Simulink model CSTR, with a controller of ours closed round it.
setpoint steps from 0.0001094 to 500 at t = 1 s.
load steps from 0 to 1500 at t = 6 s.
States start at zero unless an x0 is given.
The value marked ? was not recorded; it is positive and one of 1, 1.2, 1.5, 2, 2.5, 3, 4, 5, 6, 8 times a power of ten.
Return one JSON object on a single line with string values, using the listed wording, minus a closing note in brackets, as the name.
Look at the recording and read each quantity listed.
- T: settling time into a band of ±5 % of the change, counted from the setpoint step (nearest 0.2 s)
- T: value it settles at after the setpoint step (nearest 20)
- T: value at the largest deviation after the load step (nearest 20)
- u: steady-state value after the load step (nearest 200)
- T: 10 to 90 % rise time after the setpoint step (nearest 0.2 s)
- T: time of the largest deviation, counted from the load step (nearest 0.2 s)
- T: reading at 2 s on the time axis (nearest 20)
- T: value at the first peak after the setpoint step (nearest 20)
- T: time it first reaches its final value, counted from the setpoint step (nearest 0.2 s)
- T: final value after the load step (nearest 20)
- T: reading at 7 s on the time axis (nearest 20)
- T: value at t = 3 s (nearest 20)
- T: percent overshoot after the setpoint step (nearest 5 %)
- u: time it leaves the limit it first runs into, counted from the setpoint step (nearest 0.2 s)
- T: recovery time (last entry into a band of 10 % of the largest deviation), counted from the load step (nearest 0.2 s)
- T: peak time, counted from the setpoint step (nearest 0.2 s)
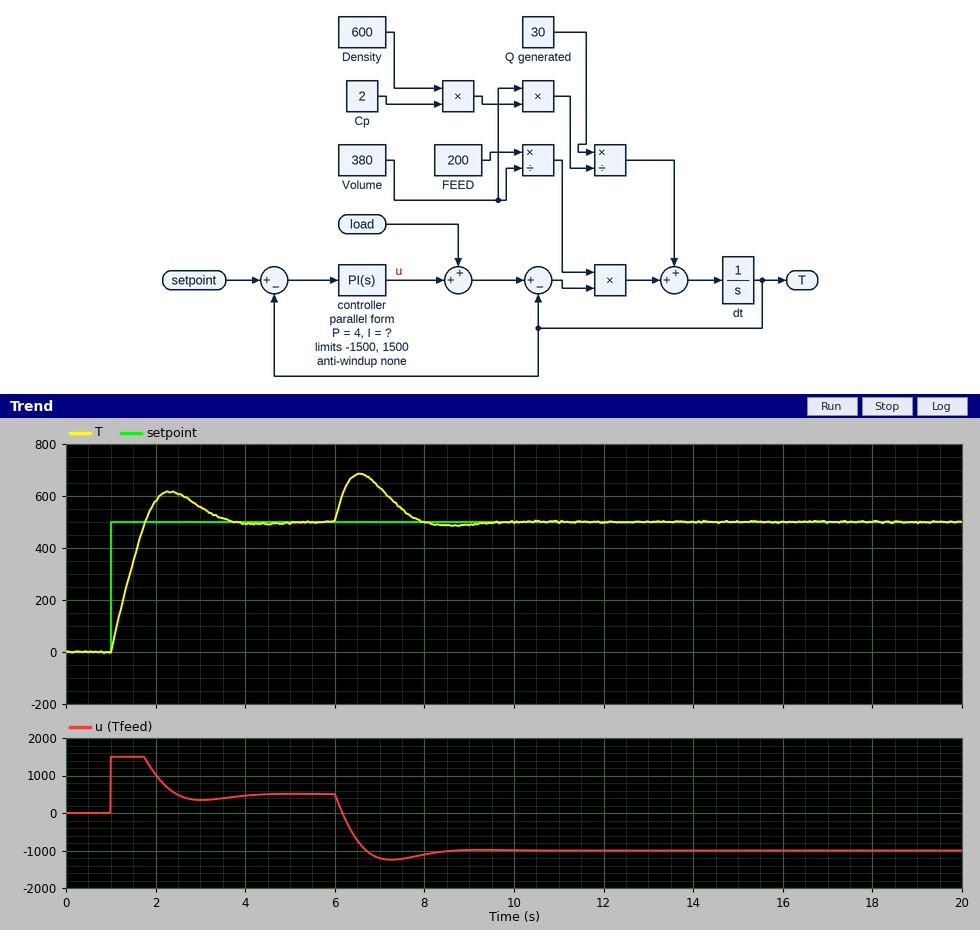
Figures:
{"T: settling time into a band of ±5 % of the change, counted from the setpoint step": "2.4 s", "T: value it settles at after the setpoint step": "500", "T: value at the largest deviation after the load step": "680", "u: steady-state value after the load step": "-1000", "T: 10 to 90 % rise time after the setpoint step": "0.6 s", "T: time of the largest deviation, counted from the load step": "0.6 s", "T: reading at 2 s on the time axis": "580", "T: value at the first peak after the setpoint step": "620", "T: time it first reaches its final value, counted from the setpoint step": "0.8 s", "T: final value after the load step": "500", "T: reading at 7 s on the time axis": "640", "T: value at t = 3 s": "560", "T: percent overshoot after the setpoint step": "25 %", "u: time it leaves the limit it first runs into, counted from the setpoint step": "0.8 s", "T: recovery time (last entry into a band of 10 % of the largest deviation), counted from the load step": "1.8 s", "T: peak time, counted from the setpoint step": "1.4 s"}
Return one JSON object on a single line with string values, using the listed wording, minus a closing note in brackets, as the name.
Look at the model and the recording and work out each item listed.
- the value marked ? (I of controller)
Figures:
{"the value marked ?": "8"}
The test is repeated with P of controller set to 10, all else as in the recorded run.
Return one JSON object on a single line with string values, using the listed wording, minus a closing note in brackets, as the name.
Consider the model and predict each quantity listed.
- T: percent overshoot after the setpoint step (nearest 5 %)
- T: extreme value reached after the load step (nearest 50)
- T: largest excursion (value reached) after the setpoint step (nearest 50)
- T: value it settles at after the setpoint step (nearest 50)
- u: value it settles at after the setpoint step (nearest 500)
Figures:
{"T: percent overshoot after the setpoint step": "15 %", "T: extreme value reached after the load step": "600", "T: largest excursion (value reached) after the setpoint step": "550", "T: value it settles at after the setpoint step": "500", "u: value it settles at after the setpoint step": "500"}
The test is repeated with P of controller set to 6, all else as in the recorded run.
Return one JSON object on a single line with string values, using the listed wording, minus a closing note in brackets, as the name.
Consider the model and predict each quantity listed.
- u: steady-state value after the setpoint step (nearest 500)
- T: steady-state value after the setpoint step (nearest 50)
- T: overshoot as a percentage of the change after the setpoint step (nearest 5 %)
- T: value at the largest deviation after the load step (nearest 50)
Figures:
{"u: steady-state value after the setpoint step": "500", "T: steady-state value after the setpoint step": "500", "T: overshoot as a percentage of the change after the setpoint step": "20 %", "T: value at the largest deviation after the load step": "650"}
